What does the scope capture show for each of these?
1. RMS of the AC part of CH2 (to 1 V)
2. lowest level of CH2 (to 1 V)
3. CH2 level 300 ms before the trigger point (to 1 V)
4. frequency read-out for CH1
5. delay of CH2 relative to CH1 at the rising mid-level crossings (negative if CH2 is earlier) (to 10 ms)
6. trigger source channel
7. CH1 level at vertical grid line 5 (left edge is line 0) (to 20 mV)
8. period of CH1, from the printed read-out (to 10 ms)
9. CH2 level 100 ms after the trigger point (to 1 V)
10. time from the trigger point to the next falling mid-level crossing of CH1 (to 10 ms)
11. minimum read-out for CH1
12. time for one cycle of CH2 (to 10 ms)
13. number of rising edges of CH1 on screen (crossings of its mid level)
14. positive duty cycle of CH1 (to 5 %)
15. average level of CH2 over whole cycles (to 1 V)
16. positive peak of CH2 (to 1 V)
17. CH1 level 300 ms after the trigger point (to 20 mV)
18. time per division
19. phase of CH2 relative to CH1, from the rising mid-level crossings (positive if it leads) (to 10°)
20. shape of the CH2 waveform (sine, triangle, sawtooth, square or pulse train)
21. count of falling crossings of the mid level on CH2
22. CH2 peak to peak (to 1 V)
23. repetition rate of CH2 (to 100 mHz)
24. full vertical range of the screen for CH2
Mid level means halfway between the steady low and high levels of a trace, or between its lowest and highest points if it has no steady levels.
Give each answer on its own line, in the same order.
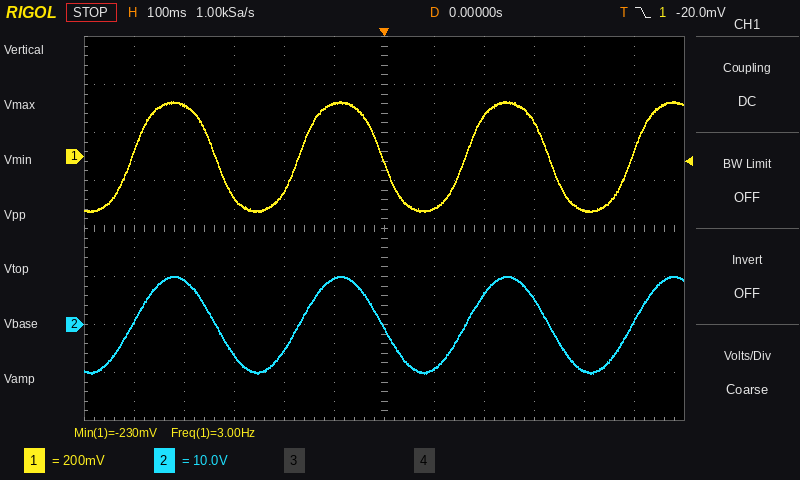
7 V
-10 V
-6 V
3.00 Hz
0 ms
CH1
220 mV
330 ms
-9 V
330 ms
-230 mV
330 ms
4
50 %
0 V
10 V
140 mV
100 ms
0°
sine
3
20 V
3.0 Hz
80 V
